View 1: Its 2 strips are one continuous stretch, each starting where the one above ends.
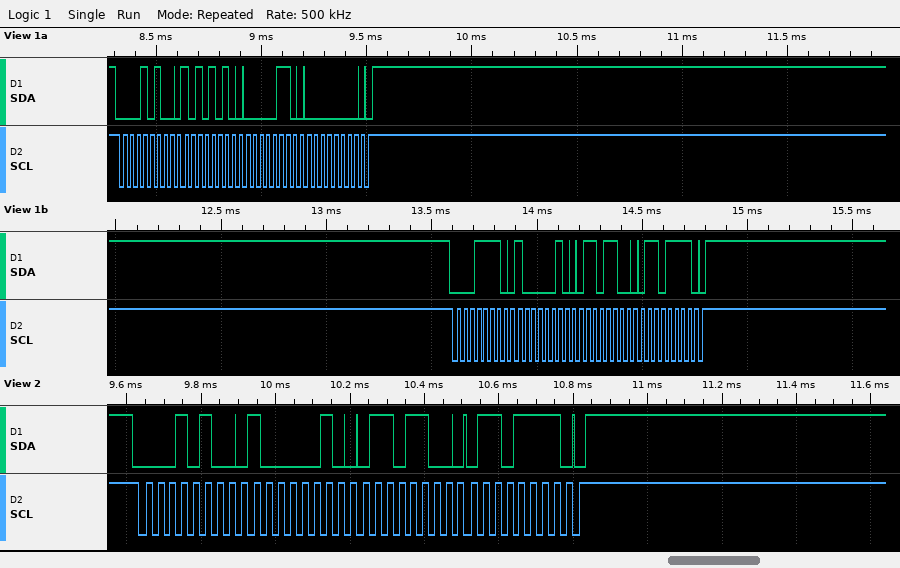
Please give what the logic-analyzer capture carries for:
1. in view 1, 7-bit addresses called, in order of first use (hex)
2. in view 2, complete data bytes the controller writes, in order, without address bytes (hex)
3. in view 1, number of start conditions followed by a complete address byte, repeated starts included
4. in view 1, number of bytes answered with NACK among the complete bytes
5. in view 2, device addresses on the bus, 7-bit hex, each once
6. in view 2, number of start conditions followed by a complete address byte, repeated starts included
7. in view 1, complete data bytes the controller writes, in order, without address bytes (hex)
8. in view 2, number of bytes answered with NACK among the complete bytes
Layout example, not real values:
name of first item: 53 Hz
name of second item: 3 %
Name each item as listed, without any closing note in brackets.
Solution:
in view 1, 7-bit addresses called, in order of first use: 0x0A 0x0F
in view 2, complete data bytes the controller writes, in order, without address bytes: 82 6C 6F
in view 1, number of start conditions followed by a complete address byte, repeated starts included: 2
in view 1, number of bytes answered with NACK among the complete bytes: 0
in view 2, device addresses on the bus, 7-bit hex, each once: 0x0A
in view 2, number of start conditions followed by a complete address byte, repeated starts included: 1
in view 1, complete data bytes the controller writes, in order, without address bytes: AA 06 00 82 6C 6F
in view 2, number of bytes answered with NACK among the complete bytes: 0
